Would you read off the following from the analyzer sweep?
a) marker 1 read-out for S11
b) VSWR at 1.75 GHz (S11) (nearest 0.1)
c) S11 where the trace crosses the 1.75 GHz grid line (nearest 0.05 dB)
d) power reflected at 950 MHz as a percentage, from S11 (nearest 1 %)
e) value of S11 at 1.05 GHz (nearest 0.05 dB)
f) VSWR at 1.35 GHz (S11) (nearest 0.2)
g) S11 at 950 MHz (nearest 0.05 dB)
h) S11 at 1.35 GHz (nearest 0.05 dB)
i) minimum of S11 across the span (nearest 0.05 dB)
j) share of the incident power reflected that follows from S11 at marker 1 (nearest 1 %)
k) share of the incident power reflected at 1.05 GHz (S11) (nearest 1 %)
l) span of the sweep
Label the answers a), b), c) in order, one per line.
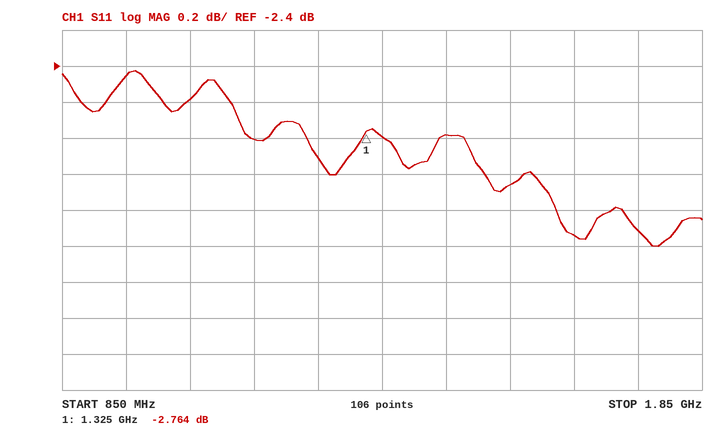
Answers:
a) -2.764 dB
b) 5.3
c) -3.30 dB
d) 57 %
e) -2.60 dB
f) 6.2
g) -2.45 dB
h) -2.80 dB
i) -3.40 dB
j) 53 %
k) 55 %
l) 1 GHz
